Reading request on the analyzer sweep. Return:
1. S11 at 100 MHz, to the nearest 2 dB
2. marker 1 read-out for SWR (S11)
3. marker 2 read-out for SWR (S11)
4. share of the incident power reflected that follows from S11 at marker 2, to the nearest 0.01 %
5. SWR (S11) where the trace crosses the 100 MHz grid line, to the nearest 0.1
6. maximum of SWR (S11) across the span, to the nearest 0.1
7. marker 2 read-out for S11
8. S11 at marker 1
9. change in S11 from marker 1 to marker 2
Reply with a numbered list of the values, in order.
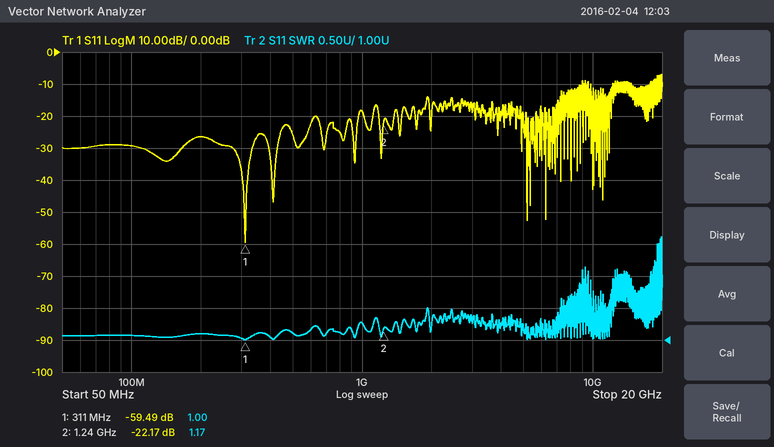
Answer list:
1. -30 dB
2. 1.00
3. 1.17
4. 0.61 %
5. 1.1
6. 2.6
7. -22.17 dB
8. -59.49 dB
9. 37.32 dB
